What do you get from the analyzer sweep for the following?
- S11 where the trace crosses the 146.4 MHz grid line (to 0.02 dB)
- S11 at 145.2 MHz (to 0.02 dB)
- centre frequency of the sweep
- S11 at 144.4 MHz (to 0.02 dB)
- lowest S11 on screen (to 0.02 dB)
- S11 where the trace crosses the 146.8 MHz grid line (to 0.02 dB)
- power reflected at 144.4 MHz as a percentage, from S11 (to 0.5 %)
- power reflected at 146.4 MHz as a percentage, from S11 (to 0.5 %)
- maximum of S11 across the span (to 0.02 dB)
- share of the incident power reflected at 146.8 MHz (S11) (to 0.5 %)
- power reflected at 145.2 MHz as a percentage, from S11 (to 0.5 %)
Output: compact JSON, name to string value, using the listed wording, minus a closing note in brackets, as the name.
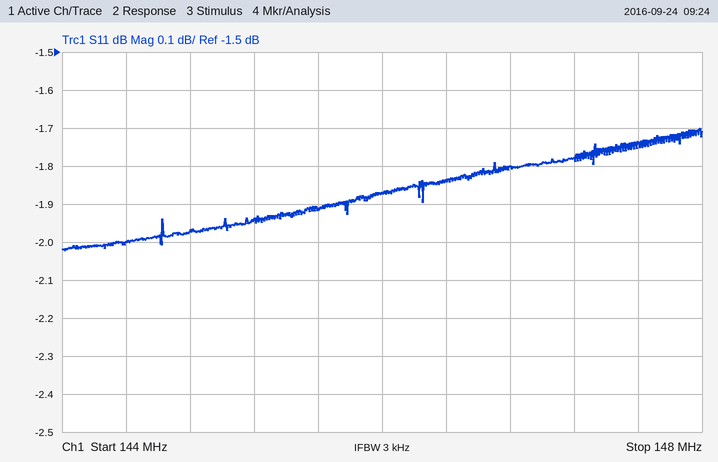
{"S11 where the trace crosses the 146.4 MHz grid line": "-1.84 dB", "S11 at 145.2 MHz": "-1.94 dB", "centre frequency of the sweep": "146 MHz", "S11 at 144.4 MHz": "-2.00 dB", "lowest S11 on screen": "-2.02 dB", "S11 where the trace crosses the 146.8 MHz grid line": "-1.80 dB", "power reflected at 144.4 MHz as a percentage, from S11": "63.0 %", "power reflected at 146.4 MHz as a percentage, from S11": "65.5 %", "maximum of S11 across the span": "-1.70 dB", "share of the incident power reflected at 146.8 MHz (S11)": "66.0 %", "power reflected at 145.2 MHz as a percentage, from S11": "64.0 %"}
